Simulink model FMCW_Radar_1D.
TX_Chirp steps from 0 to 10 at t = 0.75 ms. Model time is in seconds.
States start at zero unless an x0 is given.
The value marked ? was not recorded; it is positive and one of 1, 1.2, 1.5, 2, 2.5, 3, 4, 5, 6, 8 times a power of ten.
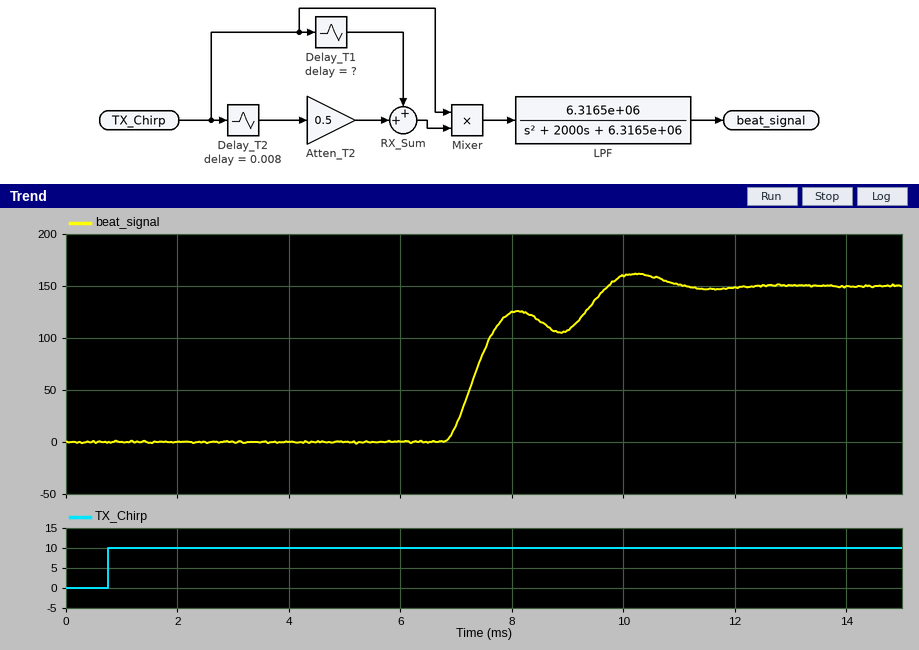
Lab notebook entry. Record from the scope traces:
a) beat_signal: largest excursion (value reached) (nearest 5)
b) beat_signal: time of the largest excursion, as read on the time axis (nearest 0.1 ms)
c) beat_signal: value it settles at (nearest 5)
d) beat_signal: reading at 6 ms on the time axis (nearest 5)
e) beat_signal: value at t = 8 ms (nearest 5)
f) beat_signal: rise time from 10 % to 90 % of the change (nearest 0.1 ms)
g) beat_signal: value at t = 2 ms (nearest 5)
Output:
160
10.2 ms
150
0
125
2.5 ms
0
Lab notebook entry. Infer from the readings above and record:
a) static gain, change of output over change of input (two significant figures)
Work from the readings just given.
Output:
15
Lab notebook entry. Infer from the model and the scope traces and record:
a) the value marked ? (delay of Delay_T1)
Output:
0.006
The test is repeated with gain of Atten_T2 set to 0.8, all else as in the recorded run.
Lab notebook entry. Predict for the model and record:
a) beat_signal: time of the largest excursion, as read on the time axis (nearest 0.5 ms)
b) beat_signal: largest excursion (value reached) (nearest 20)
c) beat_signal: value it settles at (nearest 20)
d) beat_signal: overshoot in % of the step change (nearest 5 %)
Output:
10.0 ms
200
180
10 %
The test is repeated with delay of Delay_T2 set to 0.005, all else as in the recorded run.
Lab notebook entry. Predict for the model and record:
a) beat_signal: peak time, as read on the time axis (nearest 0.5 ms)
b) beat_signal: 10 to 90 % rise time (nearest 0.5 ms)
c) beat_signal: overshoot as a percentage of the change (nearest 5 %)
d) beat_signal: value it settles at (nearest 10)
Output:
8.0 ms
1.5 ms
15 %
150
